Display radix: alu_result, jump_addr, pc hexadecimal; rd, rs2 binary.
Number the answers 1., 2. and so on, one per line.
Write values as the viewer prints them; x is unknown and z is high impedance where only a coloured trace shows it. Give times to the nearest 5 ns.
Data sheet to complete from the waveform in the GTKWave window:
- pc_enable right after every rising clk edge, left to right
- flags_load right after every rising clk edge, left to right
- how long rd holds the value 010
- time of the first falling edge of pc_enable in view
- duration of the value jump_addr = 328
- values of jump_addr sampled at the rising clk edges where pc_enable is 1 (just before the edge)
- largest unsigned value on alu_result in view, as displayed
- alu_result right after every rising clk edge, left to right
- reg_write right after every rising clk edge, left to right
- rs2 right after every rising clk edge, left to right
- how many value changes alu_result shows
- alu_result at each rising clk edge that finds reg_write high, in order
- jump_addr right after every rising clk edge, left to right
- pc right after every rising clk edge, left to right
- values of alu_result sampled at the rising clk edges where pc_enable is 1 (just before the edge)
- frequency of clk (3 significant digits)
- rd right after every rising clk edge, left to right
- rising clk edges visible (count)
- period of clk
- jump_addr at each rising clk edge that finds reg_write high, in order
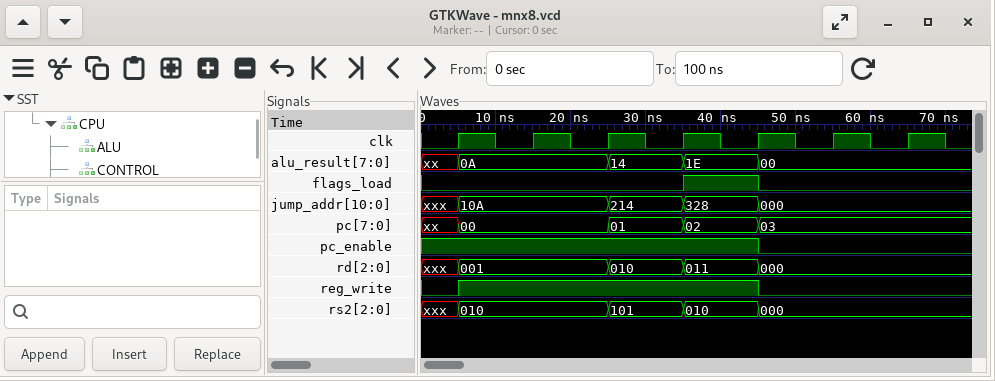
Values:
1. 1 1 1 1 0 0 0
2. 0 0 0 1 0 0 0
3. 10 ns
4. 45 ns
5. 10 ns
6. xxx, 10A, 10A, 214, 328
7. 1E
8. 0A, 0A, 14, 1E, 00, 00, 00
9. 1 1 1 1 0 0 0
10. 010, 010, 101, 010, 000, 000, 000
11. 4
12. 0A, 0A, 14, 1E
13. 10A, 10A, 214, 328, 000, 000, 000
14. 00, 00, 01, 02, 03, 03, 03
15. xx, 0A, 0A, 14, 1E
16. 100 MHz
17. 001, 001, 010, 011, 000, 000, 000
18. 7
19. 10 ns
20. 10A, 10A, 214, 328
